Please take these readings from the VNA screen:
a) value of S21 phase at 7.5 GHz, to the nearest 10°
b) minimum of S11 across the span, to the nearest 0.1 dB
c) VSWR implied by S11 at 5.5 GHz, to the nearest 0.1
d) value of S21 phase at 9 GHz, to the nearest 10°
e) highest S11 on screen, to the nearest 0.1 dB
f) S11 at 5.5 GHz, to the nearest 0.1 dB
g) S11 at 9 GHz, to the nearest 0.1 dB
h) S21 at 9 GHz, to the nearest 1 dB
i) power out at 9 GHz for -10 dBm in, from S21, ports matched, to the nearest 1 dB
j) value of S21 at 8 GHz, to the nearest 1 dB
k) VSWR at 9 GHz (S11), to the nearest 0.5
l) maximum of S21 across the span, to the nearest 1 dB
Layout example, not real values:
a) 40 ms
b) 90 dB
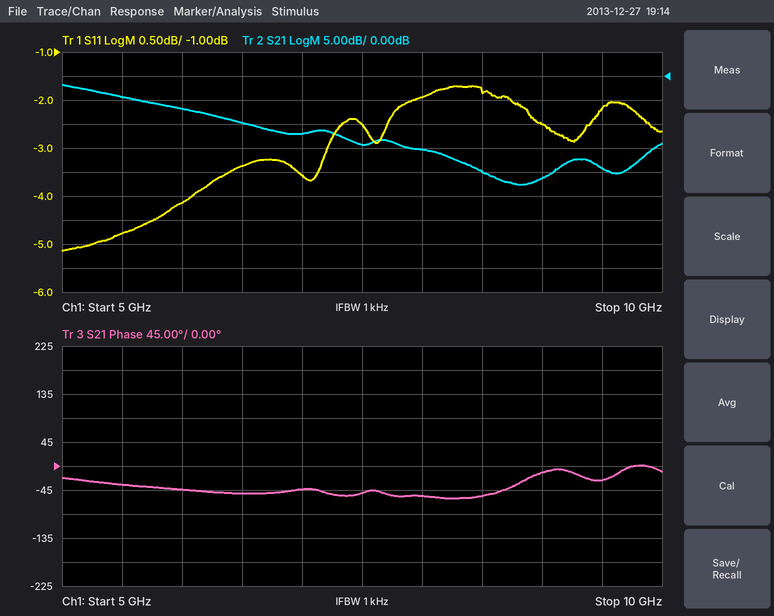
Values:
a) -50°
b) -5.1 dB
c) 3.7
d) -10°
e) -1.7 dB
f) -4.8 dB
g) -2.5 dB
h) -21 dB
i) -31 dBm
j) -15 dB
k) 7.0
l) -2 dB
